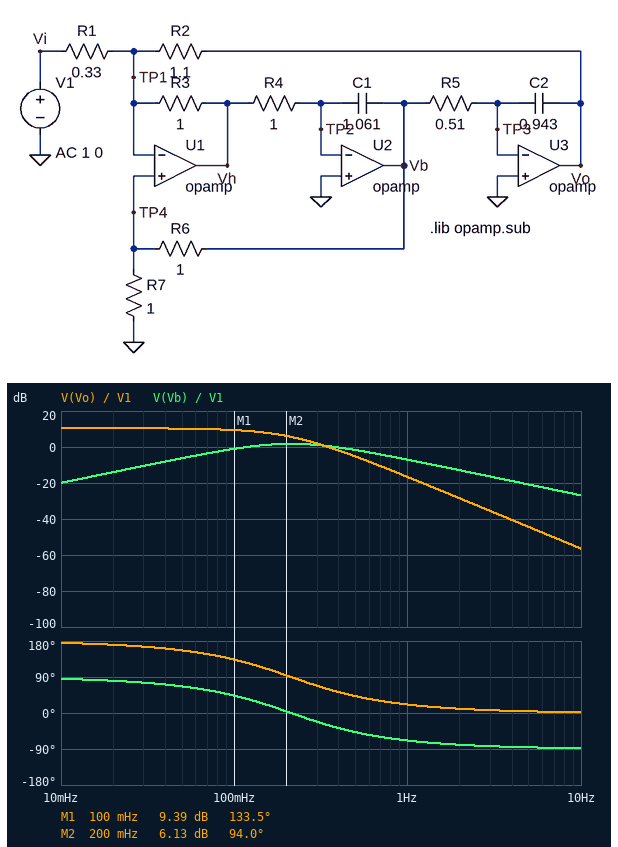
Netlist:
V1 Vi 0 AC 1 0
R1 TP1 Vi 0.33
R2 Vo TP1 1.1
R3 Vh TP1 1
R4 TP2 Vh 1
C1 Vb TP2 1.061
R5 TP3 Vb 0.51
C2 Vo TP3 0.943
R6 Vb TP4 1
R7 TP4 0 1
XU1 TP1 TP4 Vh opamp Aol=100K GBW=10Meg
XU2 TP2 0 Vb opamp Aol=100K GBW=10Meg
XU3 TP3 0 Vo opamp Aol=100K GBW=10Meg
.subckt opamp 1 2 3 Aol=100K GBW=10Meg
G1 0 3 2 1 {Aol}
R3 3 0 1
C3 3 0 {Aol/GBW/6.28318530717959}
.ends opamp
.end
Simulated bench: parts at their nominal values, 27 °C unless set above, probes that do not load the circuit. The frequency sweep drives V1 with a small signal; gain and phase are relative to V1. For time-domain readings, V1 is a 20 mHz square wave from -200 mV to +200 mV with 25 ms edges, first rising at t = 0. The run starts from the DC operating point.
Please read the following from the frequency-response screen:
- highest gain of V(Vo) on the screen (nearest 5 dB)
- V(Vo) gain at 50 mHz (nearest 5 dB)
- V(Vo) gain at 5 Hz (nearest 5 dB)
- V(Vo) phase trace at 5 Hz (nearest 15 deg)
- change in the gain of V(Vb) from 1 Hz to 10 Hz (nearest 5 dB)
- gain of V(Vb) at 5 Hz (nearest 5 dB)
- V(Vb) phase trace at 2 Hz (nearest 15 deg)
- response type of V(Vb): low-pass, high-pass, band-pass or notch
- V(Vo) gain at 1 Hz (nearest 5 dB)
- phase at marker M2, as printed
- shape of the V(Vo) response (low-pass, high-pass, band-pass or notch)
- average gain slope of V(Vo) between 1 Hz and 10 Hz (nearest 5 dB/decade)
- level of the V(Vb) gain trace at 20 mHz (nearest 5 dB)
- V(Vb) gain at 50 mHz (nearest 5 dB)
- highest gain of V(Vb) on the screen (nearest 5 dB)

10 dB
10 dB
-45 dB
0 deg
-20 dB
-20 dB
-75 deg
band-pass
-15 dB
94.0 deg
low-pass
-40 dB/decade
-15 dB
-5 dB
0 dB
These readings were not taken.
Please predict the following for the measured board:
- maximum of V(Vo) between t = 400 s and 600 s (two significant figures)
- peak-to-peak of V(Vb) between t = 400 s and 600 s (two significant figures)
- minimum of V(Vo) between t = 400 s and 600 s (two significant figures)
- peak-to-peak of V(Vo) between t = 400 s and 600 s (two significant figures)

670 mV
690 mV
-670 mV
1.3 V
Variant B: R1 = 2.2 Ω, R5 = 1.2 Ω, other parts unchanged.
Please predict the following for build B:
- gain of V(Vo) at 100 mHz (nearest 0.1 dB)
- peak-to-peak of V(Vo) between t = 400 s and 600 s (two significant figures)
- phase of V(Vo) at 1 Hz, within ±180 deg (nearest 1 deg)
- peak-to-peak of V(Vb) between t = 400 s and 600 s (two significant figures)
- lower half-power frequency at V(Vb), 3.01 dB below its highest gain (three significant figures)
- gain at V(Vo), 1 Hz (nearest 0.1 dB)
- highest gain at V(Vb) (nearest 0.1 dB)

-6.4 dB
230 mV
10 deg
190 mV
75.8 mHz
-40.3 dB
-8.3 dB
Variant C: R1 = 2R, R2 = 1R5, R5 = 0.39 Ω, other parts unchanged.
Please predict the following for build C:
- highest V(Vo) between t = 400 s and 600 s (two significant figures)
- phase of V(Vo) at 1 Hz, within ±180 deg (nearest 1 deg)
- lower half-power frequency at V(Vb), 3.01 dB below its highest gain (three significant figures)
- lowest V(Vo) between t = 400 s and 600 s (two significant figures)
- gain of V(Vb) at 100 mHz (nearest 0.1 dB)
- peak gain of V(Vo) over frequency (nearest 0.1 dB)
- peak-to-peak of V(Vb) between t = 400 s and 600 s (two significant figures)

230 mV
10 deg
142 mHz
-230 mV
-13.9 dB
0.4 dB
180 mV
